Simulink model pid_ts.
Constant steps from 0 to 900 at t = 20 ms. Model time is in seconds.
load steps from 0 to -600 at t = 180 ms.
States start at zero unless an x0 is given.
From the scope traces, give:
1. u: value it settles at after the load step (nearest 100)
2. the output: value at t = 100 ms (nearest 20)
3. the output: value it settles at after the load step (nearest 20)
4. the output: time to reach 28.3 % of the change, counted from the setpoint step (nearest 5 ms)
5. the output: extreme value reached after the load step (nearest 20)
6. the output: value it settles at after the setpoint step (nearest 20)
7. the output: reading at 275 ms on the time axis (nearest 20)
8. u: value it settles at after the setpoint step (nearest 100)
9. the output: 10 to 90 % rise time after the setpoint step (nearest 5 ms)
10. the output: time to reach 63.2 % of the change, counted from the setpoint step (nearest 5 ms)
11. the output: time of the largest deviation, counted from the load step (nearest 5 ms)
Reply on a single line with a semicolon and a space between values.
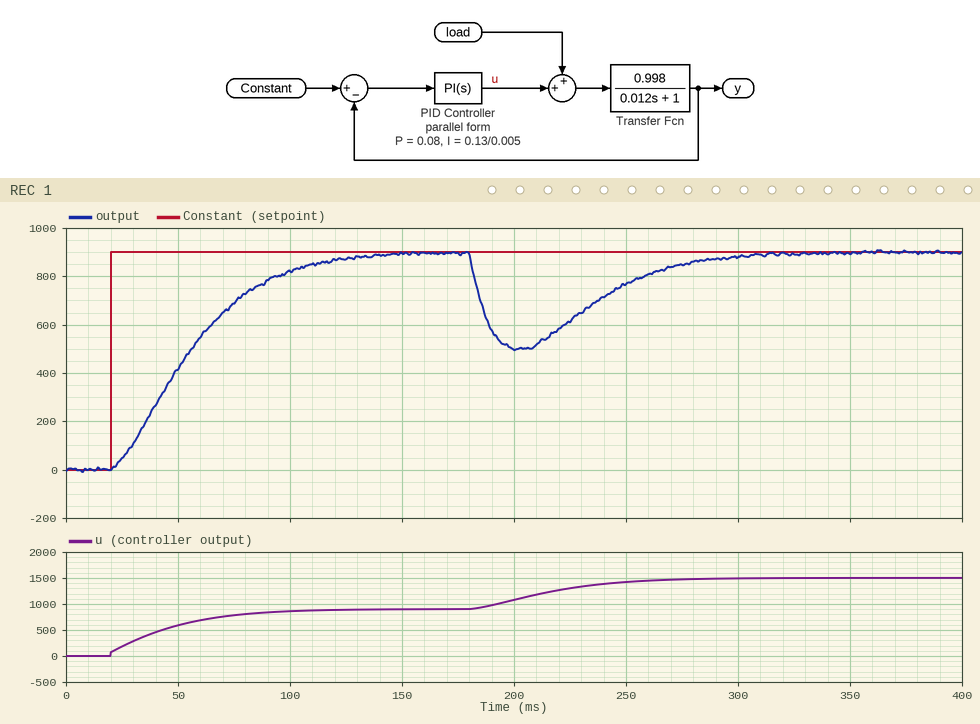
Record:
1500; 820; 900; 20 ms; 500; 900; 840; 900; 70 ms; 40 ms; 20 ms
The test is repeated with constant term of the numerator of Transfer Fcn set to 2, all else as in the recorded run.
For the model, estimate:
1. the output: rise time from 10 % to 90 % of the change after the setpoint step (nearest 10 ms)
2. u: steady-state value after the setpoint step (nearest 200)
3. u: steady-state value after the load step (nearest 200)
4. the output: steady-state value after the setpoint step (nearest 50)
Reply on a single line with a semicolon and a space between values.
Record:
30 ms; 400; 1000; 900
